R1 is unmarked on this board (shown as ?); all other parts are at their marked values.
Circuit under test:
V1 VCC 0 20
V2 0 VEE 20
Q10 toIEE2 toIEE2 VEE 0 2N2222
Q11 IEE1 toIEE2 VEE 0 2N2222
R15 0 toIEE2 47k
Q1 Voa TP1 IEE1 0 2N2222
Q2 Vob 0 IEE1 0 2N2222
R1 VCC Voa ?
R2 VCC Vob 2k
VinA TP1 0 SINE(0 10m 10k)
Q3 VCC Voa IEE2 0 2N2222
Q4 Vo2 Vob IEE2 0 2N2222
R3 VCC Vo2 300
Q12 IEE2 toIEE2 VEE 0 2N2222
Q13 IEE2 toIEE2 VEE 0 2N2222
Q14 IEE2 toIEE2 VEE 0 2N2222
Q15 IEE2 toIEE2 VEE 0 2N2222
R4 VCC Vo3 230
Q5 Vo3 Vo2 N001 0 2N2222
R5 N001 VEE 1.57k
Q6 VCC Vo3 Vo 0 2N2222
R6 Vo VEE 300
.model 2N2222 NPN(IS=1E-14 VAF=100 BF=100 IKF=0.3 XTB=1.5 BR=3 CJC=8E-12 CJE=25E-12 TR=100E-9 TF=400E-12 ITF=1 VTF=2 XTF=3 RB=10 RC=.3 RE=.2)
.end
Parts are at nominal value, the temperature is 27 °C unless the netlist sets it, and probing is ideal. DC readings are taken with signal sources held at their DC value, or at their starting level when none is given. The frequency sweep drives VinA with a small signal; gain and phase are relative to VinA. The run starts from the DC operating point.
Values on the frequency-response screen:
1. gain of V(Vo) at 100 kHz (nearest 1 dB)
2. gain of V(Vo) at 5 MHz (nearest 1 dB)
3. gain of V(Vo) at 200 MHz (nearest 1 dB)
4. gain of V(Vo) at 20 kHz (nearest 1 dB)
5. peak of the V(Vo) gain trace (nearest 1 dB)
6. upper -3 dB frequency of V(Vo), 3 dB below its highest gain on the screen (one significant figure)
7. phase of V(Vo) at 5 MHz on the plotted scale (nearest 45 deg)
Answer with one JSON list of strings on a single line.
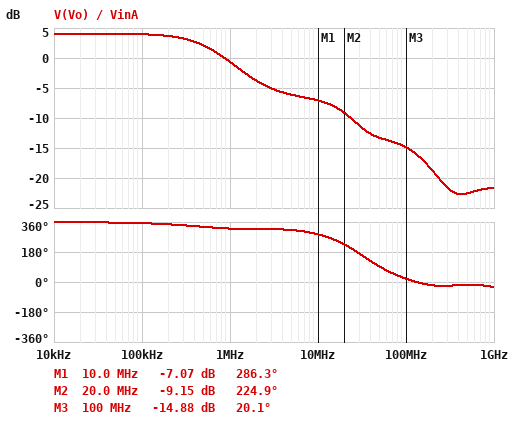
["4 dB", "-6 dB", "-19 dB", "4 dB", "4 dB", "700 kHz", "315 deg"]
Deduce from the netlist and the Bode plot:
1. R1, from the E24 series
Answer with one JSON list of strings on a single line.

["910 Ω"]
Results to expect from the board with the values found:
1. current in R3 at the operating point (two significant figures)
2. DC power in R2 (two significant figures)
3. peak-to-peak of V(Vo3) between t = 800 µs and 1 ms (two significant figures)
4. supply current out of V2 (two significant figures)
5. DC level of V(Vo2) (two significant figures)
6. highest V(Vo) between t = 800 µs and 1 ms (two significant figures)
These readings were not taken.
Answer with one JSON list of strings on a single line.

["8.1 mA", "1.5 mW", "32 mV", "150 mA", "18 V", "16 V"]
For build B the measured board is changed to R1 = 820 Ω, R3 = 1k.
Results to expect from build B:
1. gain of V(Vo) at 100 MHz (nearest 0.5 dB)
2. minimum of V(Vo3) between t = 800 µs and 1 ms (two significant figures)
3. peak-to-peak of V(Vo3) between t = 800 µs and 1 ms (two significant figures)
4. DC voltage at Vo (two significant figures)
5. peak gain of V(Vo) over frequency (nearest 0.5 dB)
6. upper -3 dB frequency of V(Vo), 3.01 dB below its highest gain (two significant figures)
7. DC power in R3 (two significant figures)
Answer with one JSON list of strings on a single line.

["-14.5 dB", "16 V", "41 mV", "15 V", "6.5 dB", "720 kHz", "10 mW"]
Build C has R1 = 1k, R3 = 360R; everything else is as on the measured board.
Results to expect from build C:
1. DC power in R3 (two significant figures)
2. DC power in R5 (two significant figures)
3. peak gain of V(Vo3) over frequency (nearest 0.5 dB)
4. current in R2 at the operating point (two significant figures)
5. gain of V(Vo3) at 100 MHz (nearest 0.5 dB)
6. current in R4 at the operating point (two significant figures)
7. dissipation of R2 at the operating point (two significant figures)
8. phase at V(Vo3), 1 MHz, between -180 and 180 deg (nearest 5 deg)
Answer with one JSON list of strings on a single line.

["18 mW", "850 mW", "4.5 dB", "950 µA", "-14.5 dB", "15 mA", "1.8 mW", "-40 deg"]
